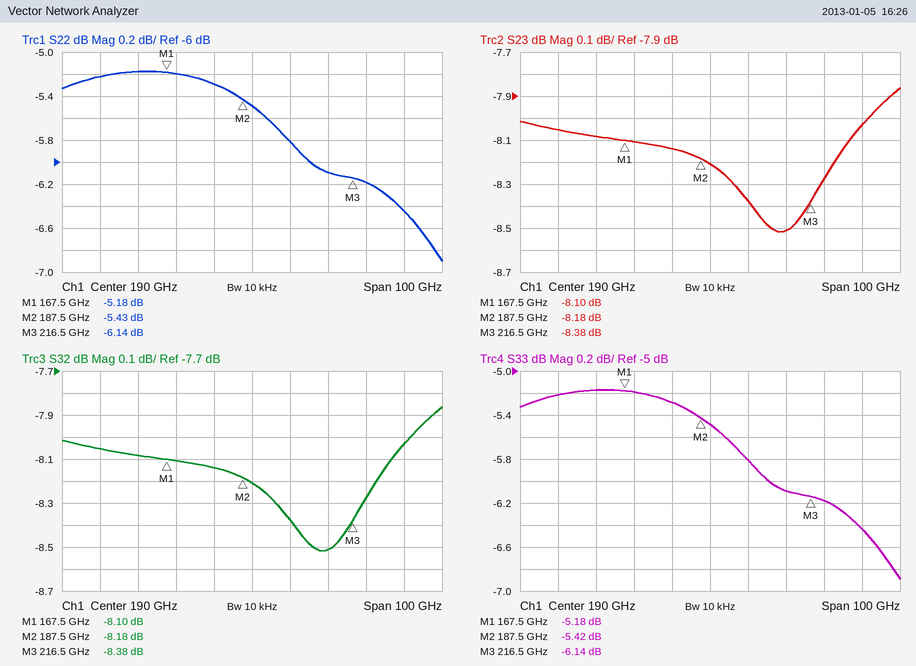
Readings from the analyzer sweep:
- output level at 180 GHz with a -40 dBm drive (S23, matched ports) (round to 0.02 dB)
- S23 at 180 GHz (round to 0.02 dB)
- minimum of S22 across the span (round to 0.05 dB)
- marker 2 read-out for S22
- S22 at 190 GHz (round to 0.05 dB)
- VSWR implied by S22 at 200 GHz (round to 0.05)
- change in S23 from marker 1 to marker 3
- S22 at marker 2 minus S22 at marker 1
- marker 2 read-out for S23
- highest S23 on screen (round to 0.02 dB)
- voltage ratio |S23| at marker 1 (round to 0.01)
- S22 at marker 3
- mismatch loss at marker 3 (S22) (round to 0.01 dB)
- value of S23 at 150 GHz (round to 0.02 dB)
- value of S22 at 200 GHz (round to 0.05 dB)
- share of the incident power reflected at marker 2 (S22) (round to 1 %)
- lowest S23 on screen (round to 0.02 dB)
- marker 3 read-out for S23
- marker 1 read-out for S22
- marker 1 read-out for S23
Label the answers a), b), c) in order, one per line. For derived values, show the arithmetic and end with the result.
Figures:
a) -40 dBm + (-8.14 dB) = -48.14 dBm
b) -8.14 dB
c) -6.90 dB
d) -5.43 dB
e) -5.50 dB
f) |Γ| = 10^(-5.8/20) = 0.5129; VSWR = (1 + 0.5129)/(1 − 0.5129) ≈ 3.11, so 3.10 to the nearest 0.05
g) -8.38 − (-8.1) = -0.28 dB
h) -5.43 − (-5.18) = -0.25 dB
i) -8.18 dB
j) -7.86 dB
k) 10^(-8.1/20) ≈ 0.39
l) -6.14 dB
m) −10 log10(1 − 10^(-6.14/10)) ≈ 1.21 dB
n) -8.06 dB
o) -5.80 dB
p) 10^(-5.43/10) ≈ 29 %
q) -8.52 dB
r) -8.38 dB
s) -5.18 dB
t) -8.10 dB
